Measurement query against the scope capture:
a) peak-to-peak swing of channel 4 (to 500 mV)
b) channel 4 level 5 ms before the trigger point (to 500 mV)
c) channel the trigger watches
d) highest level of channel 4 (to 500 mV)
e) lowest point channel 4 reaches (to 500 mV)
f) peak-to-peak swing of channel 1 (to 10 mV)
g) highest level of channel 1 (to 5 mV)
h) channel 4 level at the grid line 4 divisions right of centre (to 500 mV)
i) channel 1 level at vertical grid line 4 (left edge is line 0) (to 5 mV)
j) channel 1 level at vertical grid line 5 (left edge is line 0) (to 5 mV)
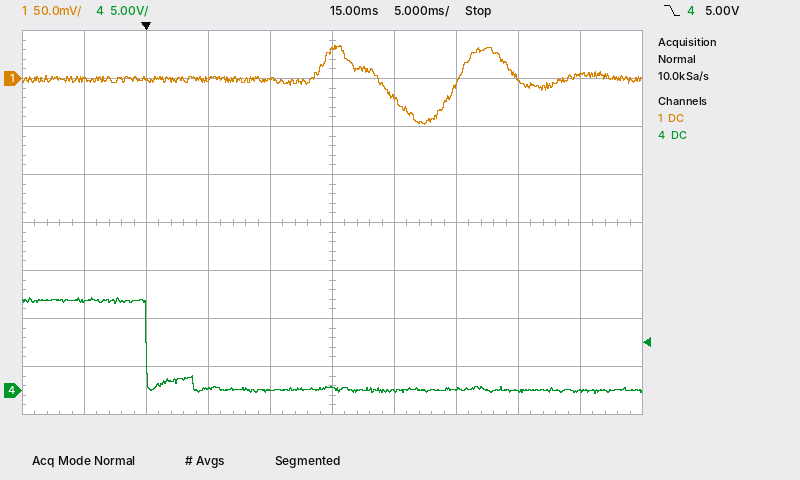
10.0 V
9.5 V
channel 4
9.5 V
-500 mV
80 mV
35 mV
0.0 V
0 mV
30 mV
